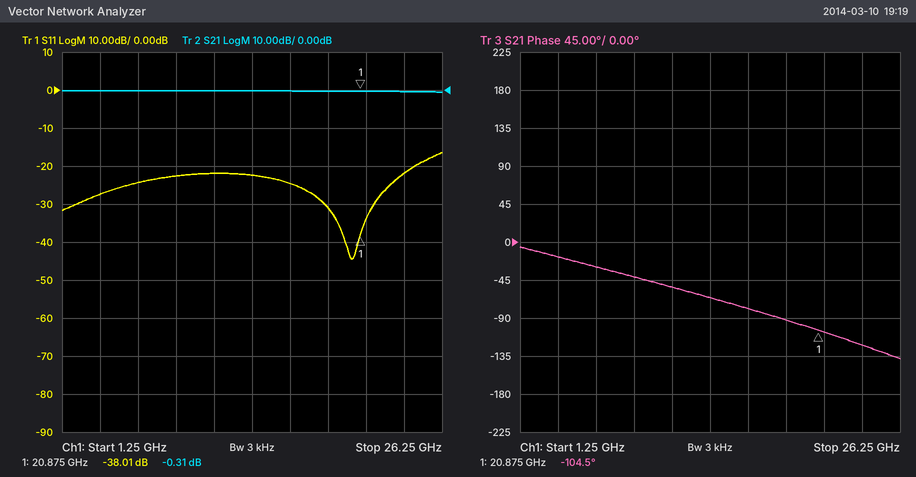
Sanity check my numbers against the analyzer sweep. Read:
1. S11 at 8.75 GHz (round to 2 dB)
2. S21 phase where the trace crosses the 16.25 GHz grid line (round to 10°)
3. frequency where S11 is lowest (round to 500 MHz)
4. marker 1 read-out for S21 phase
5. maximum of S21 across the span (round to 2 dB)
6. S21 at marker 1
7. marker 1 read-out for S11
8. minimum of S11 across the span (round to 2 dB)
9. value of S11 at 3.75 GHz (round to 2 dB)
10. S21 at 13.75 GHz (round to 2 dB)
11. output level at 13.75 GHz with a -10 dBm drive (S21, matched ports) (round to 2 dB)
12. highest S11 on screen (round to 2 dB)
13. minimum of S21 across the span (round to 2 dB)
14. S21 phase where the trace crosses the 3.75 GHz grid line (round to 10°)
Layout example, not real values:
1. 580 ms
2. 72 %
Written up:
1. -22 dB
2. -80°
3. 20.5 GHz
4. -104.5°
5. 0 dB
6. -0.31 dB
7. -38.01 dB
8. -44 dB
9. -28 dB
10. 0 dB
11. -10 dBm
12. -16 dB
13. 0 dB
14. -20°
